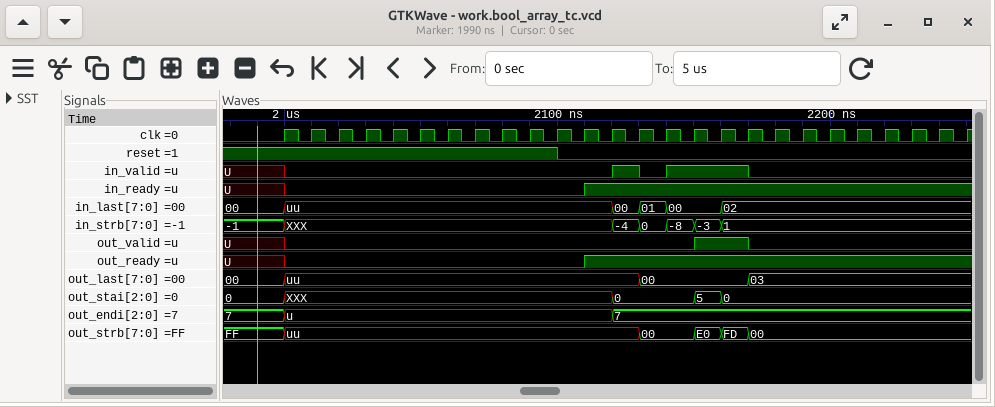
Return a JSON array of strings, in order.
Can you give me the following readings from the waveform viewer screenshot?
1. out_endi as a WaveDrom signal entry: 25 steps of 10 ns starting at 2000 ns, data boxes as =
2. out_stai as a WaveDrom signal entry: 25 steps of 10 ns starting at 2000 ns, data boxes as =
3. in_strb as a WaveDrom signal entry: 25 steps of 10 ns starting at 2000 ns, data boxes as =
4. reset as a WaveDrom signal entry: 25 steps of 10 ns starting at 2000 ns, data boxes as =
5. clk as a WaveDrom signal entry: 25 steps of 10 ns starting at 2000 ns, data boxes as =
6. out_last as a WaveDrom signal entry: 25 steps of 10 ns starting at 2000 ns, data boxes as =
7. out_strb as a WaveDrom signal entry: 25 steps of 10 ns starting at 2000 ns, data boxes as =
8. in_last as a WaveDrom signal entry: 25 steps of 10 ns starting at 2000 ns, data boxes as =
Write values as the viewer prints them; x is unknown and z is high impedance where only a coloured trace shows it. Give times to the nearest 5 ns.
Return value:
["{name: 'out_endi', wave: 'x...........=............', data: '7'}", "{name: 'out_stai', wave: 'x...........=..==........', data: '0 5 0'}", "{name: 'in_strb', wave: 'x...........=====........', data: '-4 0 -8 -3 1'}", "{name: 'reset', wave: '1.........0..............'}", "{name: 'clk', wave: 'p........................'}", "{name: 'out_last', wave: 'x............=...=.......', data: '00 03'}", "{name: 'out_strb', wave: 'x............=.===.......', data: '00 E0 FD 00'}", "{name: 'in_last', wave: 'x...........===.=........', data: '00 01 00 02'}"]
